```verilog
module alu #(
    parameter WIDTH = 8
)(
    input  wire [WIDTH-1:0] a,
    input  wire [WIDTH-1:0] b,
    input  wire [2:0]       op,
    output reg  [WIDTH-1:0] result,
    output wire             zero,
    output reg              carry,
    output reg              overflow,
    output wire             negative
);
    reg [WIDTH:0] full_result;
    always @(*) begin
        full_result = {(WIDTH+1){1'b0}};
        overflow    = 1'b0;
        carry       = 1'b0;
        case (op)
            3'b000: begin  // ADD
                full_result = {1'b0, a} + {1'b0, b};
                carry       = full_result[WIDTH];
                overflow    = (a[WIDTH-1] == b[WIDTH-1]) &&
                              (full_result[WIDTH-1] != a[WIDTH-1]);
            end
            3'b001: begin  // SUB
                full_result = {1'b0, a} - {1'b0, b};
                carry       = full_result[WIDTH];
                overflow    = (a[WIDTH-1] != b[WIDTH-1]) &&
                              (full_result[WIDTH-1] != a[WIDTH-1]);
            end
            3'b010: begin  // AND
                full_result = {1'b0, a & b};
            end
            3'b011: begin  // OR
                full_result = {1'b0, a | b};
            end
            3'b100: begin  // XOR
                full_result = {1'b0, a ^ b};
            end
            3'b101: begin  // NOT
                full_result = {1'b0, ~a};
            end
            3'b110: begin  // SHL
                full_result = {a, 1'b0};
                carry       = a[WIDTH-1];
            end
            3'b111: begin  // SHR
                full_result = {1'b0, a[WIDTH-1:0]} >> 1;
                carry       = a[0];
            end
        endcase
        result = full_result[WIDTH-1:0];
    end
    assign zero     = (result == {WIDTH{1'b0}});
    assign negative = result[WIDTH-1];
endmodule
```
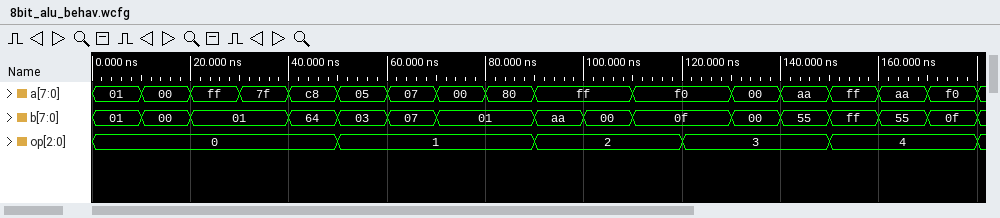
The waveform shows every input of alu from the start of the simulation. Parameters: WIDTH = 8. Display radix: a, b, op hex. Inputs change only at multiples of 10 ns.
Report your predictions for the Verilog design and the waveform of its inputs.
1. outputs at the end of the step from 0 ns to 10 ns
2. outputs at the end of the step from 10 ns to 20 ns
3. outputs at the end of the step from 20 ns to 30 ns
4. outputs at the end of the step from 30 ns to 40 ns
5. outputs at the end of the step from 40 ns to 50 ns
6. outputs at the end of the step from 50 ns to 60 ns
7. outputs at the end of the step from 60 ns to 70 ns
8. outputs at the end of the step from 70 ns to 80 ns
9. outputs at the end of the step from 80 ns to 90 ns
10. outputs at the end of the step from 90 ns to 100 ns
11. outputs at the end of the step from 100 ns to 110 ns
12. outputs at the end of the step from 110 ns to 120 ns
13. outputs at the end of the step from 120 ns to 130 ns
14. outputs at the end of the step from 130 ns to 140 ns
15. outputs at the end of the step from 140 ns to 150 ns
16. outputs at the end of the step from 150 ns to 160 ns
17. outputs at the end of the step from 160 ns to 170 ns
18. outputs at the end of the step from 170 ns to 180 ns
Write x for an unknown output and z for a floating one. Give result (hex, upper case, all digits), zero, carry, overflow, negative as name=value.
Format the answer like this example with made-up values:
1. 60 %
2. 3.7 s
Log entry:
1. result=02, zero=0, carry=0, overflow=0, negative=0
2. result=00, zero=1, carry=0, overflow=0, negative=0
3. result=00, zero=1, carry=1, overflow=0, negative=0
4. result=80, zero=0, carry=0, overflow=1, negative=1
5. result=2C, zero=0, carry=1, overflow=0, negative=0
6. result=02, zero=0, carry=0, overflow=0, negative=0
7. result=00, zero=1, carry=0, overflow=0, negative=0
8. result=FF, zero=0, carry=1, overflow=0, negative=1
9. result=7F, zero=0, carry=0, overflow=1, negative=0
10. result=AA, zero=0, carry=0, overflow=0, negative=1
11. result=00, zero=1, carry=0, overflow=0, negative=0
12. result=00, zero=1, carry=0, overflow=0, negative=0
13. result=FF, zero=0, carry=0, overflow=0, negative=1
14. result=00, zero=1, carry=0, overflow=0, negative=0
15. result=FF, zero=0, carry=0, overflow=0, negative=1
16. result=00, zero=1, carry=0, overflow=0, negative=0
17. result=FF, zero=0, carry=0, overflow=0, negative=1
18. result=FF, zero=0, carry=0, overflow=0, negative=1
